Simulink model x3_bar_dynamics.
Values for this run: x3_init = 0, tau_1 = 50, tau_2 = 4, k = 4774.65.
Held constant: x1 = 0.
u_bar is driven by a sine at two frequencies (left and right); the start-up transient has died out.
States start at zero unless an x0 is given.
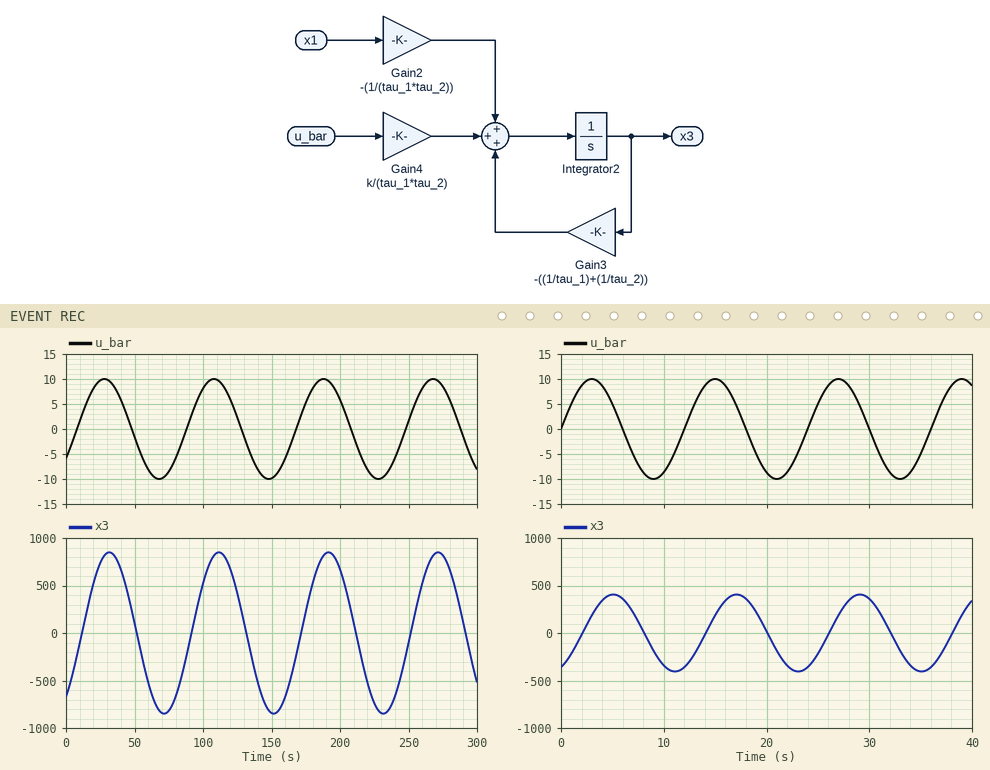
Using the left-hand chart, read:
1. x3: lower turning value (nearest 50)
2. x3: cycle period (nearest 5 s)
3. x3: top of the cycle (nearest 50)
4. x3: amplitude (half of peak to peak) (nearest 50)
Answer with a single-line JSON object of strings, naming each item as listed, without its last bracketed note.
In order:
{"x3: lower turning value": "-850", "x3: cycle period": "80 s", "x3: top of the cycle": "850", "x3: amplitude (half of peak to peak)": "850"}
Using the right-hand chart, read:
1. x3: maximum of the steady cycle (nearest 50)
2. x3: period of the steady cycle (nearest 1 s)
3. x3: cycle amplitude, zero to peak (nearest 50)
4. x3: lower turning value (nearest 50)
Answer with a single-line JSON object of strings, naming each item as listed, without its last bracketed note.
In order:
{"x3: maximum of the steady cycle": "400", "x3: period of the steady cycle": "12 s", "x3: cycle amplitude, zero to peak": "400", "x3: lower turning value": "-400"}
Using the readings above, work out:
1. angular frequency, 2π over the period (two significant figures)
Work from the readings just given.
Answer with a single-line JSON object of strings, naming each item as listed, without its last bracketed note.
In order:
{"angular frequency, 2π over the period": "0.52 rad/s"}
